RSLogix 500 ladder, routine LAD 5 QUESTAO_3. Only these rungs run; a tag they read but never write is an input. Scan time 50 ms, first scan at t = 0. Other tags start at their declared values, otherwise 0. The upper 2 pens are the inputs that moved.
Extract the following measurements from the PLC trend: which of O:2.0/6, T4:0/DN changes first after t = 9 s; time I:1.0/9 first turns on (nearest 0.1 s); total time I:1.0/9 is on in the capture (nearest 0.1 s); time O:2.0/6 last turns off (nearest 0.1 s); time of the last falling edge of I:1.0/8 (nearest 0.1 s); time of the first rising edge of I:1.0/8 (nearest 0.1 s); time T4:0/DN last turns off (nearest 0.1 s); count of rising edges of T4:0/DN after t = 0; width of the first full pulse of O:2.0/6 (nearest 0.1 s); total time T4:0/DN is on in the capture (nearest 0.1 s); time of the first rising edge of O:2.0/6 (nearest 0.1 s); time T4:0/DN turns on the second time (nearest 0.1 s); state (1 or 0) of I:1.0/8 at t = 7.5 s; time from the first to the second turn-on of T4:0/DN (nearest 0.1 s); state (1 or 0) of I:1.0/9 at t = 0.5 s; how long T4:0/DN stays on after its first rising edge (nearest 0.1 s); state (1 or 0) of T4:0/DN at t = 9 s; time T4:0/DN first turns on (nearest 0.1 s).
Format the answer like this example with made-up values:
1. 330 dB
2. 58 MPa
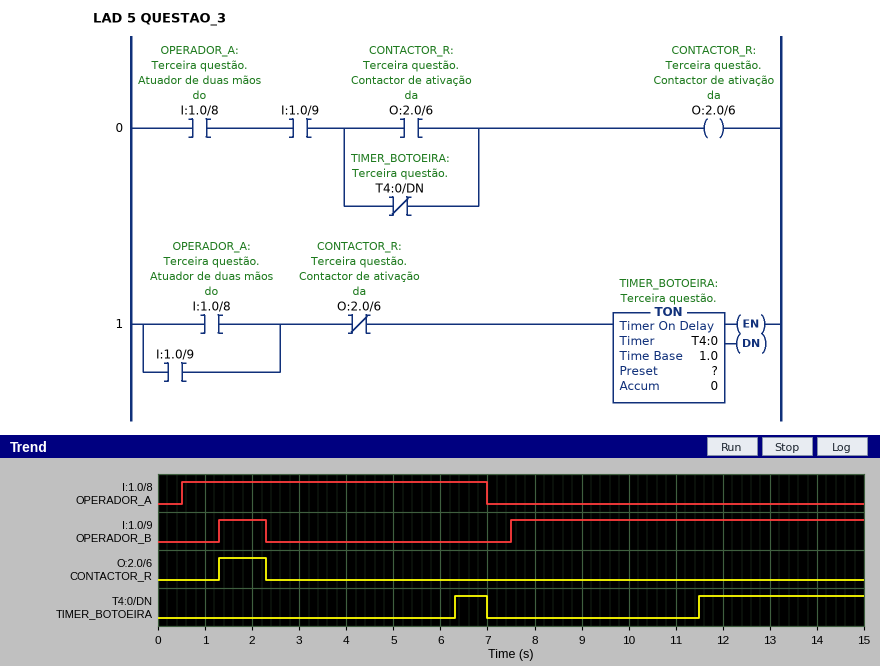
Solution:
1. T4:0/DN
2. 1.3 s
3. 8.5 s
4. 2.3 s
5. 7.0 s
6. 0.5 s
7. 7.0 s
8. 2
9. 1.0 s
10. 4.2 s
11. 1.3 s
12. 11.5 s
13. 0
14. 5.2 s
15. 0
16. 0.7 s
17. 0
18. 6.3 s
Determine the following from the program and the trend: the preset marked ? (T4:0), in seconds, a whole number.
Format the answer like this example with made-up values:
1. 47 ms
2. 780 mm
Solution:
1. 4 s
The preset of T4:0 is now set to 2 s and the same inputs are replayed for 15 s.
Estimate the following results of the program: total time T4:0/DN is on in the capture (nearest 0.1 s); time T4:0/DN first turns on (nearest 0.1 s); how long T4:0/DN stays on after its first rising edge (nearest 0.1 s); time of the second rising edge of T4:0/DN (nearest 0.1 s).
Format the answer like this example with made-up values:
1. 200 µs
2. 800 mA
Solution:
1. 8.2 s
2. 4.3 s
3. 2.7 s
4. 9.5 s
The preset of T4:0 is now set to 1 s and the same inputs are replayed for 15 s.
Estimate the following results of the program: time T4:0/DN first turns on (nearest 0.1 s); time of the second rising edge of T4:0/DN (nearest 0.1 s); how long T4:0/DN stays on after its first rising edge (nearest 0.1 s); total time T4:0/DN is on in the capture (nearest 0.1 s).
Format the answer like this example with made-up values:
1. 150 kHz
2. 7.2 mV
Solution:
1. 3.3 s
2. 8.5 s
3. 3.7 s
4. 10.2 s
